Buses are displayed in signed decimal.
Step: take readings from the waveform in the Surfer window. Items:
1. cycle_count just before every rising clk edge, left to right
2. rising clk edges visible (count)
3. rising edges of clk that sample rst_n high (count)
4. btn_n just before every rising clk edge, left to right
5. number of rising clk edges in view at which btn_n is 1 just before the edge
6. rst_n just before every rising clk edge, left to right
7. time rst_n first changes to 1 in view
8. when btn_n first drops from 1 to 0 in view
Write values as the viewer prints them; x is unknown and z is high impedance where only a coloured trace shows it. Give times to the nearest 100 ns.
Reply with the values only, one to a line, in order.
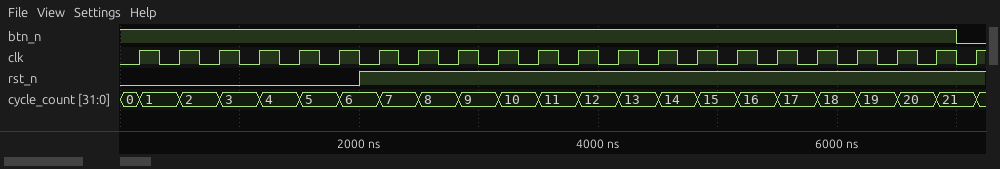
0, 1, 2, 3, 4, 5, 6, 7, 8, 9, 10, 11, 12, 13, 14, 15, 16, 17, 18, 19, 20, 21
22
16
1 1 1 1 1 1 1 1 1 1 1 1 1 1 1 1 1 1 1 1 1 0
21
0 0 0 0 0 0 1 1 1 1 1 1 1 1 1 1 1 1 1 1 1 1
2000 ns
7000 ns
